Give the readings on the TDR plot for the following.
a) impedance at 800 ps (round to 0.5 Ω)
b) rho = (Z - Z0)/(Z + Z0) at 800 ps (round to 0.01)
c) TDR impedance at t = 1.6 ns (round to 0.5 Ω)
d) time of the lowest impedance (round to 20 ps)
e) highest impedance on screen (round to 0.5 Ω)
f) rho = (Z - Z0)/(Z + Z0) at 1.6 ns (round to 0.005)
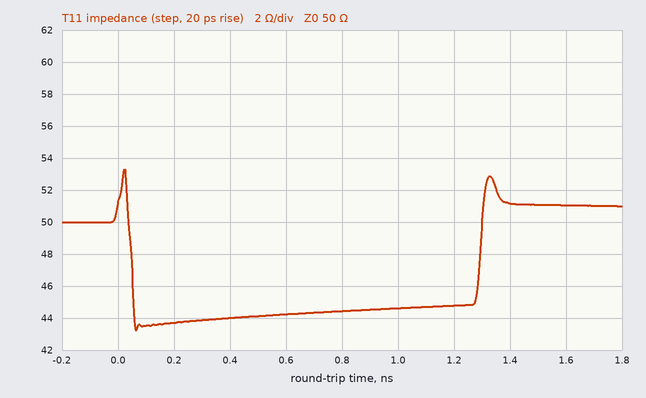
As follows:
44.5 Ω
-0.06
51.0 Ω
60 ps
53.5 Ω
+0.010
